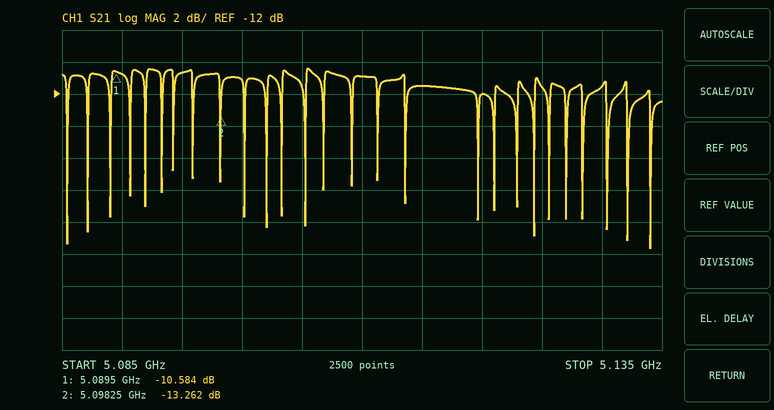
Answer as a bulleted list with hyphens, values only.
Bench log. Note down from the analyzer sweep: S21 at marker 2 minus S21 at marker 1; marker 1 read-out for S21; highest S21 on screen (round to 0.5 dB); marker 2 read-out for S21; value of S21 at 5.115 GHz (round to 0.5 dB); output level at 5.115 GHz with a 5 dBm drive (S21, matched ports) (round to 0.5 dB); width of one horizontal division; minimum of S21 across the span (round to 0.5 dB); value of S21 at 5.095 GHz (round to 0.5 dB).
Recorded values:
- -2.678 dB
- -10.584 dB
- -10.5 dB
- -13.262 dB
- -11.5 dB
- -6.5 dBm
- 5 MHz
- -21.5 dB
- -10.5 dB
